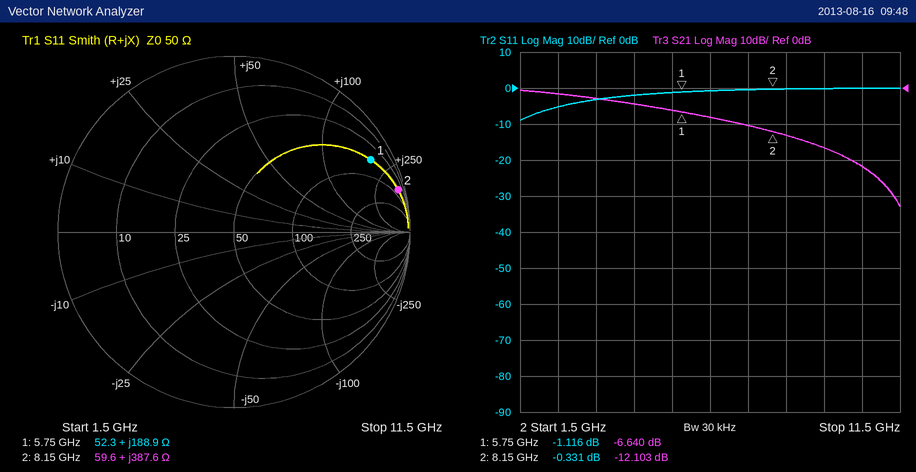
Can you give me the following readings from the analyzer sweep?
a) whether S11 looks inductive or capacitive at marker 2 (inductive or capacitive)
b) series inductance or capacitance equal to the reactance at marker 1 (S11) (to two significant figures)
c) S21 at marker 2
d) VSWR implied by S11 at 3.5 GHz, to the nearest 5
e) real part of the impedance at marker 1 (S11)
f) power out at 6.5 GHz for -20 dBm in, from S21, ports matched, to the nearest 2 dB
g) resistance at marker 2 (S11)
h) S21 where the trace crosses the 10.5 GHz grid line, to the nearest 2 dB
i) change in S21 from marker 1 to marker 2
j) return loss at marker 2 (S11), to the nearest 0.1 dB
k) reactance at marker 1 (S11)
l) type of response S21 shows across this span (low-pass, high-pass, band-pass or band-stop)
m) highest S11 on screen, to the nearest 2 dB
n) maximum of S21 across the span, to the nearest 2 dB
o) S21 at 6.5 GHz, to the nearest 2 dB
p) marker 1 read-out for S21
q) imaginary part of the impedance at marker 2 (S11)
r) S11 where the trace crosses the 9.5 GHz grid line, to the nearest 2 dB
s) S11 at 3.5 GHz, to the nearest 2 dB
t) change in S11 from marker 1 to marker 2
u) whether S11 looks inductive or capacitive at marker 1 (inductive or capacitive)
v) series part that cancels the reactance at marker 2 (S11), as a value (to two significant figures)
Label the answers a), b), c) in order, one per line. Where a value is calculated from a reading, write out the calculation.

a) inductive
b) L = 188.9 Ω/(2π × 5.75 GHz) ≈ 5.2 nH
c) -12.103 dB
d) |Γ| = 10^(-4/20) = 0.6310; VSWR = (1 + 0.6310)/(1 − 0.6310) ≈ 4.42, so 5 to the nearest 5
e) 52.3 Ω
f) -20 dBm + (-8 dB) = -28 dBm
g) 59.6 Ω
h) -22 dB
i) -12.103 − (-6.64) = -5.463 dB
j) 0.3 dB
k) +188.9 Ω
l) low-pass
m) 0 dB
n) 0 dB
o) -8 dB
p) -6.640 dB
q) +387.6 Ω
r) 0 dB
s) -4 dB
t) -0.331 − (-1.116) = 0.785 dB
u) inductive
v) C = 1/(2π × 8.15 GHz × 387.6 Ω) ≈ 50 fF
